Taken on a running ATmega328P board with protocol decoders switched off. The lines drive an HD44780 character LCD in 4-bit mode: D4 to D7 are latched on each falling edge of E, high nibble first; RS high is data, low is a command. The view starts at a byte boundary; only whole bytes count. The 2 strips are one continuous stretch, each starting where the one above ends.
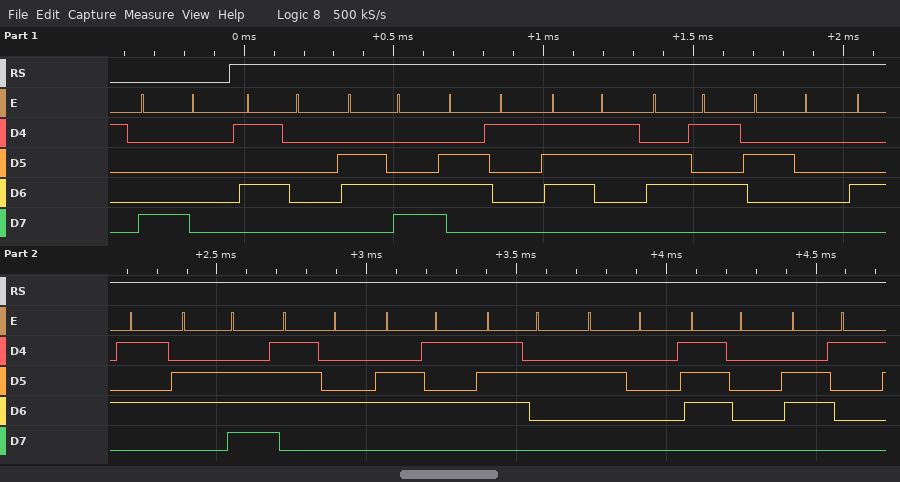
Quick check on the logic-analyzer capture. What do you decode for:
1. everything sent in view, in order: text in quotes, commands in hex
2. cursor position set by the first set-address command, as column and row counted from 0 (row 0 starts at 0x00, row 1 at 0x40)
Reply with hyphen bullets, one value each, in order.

- 0x80 "Plase Enter pa"
- column 0, row 0
